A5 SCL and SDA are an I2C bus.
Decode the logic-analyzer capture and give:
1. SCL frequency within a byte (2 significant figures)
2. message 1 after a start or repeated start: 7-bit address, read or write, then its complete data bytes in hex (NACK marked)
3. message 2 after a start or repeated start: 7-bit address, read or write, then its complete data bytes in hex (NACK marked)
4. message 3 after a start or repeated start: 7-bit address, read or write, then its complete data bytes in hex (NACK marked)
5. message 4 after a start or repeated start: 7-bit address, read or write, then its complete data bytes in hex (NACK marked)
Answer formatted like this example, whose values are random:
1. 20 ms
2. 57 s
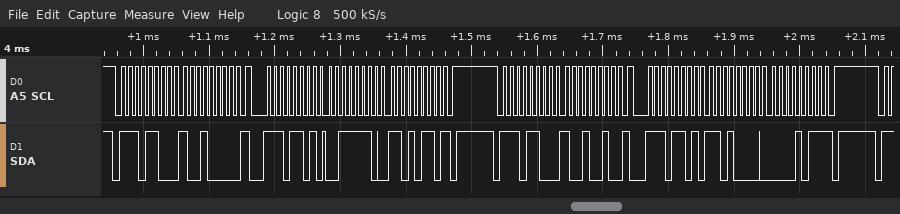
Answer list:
1. 100 kHz
2. 0x76 write: 90
3. 0x76 read: 3E D6 NACK
4. 0x76 write: 92
5. 0x76 read: D0 0B NACK
